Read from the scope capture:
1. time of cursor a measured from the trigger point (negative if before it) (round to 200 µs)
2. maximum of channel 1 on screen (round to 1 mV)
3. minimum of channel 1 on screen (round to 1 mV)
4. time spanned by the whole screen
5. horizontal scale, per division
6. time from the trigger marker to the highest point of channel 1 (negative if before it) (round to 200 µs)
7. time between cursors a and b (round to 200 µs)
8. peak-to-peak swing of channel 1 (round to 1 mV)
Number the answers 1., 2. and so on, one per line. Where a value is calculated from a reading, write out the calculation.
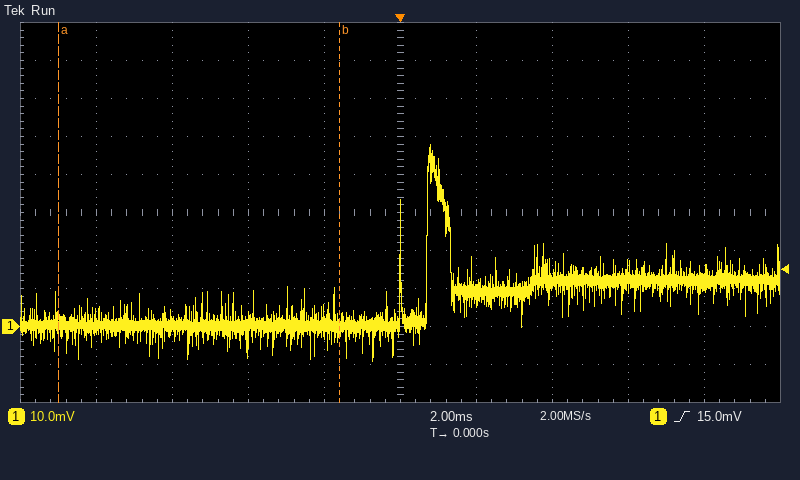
1. -9.0 ms
2. 48 mV
3. -9 mV
4. 20 ms
5. 2 ms
6. +800 µs
7. 7.4 ms
8. 48 mV − (-9 mV) = 57 mV
